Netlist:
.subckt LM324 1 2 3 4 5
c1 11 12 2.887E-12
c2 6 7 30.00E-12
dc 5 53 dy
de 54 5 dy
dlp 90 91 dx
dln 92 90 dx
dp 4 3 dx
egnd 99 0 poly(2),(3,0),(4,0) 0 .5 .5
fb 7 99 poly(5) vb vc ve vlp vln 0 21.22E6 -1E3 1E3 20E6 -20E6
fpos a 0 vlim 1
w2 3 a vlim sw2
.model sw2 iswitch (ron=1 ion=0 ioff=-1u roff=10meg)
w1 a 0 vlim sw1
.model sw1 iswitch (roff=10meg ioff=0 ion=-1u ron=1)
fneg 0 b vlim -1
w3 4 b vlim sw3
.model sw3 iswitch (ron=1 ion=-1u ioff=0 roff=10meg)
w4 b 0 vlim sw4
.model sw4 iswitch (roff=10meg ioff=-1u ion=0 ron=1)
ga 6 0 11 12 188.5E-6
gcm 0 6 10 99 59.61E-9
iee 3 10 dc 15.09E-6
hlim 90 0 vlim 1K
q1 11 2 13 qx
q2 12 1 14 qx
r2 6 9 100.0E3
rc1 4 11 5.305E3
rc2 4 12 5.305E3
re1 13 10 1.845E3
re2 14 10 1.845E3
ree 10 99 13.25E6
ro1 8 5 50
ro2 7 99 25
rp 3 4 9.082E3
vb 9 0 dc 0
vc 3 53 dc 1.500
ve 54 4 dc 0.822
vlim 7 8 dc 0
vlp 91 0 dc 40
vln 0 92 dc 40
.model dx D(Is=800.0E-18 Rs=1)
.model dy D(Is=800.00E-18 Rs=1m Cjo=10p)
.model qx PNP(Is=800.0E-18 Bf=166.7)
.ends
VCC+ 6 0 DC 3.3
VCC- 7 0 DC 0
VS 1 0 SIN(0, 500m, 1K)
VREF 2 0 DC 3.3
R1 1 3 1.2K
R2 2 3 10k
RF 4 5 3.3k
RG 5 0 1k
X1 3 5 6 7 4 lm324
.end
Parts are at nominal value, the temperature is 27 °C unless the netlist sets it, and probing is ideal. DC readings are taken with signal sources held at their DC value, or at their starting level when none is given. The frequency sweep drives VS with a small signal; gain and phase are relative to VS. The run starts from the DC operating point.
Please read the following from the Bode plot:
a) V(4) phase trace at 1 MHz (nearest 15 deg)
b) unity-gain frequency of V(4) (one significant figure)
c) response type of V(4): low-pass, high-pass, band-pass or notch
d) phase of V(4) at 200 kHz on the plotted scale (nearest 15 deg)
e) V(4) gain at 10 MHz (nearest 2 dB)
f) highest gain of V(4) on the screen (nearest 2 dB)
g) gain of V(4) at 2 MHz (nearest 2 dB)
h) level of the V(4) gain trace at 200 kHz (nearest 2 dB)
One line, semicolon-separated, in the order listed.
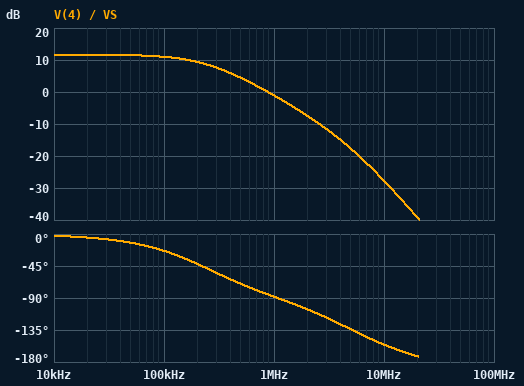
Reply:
-90 deg; 900 kHz; low-pass; -45 deg; -28 dB; 12 dB; -8 dB; 10 dB
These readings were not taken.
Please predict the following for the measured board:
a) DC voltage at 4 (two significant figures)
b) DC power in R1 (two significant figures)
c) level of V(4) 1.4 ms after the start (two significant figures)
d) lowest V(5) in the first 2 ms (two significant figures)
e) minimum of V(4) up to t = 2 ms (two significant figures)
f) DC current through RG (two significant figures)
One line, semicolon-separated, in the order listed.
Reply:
1.5 V; 100 µW; 2.6 V; 1.3 mV; 5.7 mV; 350 µA
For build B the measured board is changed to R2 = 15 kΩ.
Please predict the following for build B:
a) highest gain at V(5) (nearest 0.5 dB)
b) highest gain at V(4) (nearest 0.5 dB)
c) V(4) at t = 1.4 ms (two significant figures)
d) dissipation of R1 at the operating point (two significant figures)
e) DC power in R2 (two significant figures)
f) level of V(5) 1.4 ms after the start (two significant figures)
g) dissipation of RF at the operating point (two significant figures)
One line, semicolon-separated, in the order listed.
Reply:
-0.5 dB; 12.0 dB; 2.2 V; 50 µW; 620 µW; 520 mV; 200 µW
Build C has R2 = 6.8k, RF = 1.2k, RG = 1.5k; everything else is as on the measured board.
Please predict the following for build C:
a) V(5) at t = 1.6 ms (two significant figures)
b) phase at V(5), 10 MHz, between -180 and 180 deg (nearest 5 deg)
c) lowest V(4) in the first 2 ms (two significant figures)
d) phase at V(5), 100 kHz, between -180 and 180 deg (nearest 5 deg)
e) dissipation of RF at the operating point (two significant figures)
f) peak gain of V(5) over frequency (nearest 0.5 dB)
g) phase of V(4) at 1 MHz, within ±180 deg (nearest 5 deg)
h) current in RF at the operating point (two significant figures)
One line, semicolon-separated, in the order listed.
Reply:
250 mV; -155 deg; 130 mV; -10 deg; 130 µW; -1.5 dB; -70 deg; 330 µA
